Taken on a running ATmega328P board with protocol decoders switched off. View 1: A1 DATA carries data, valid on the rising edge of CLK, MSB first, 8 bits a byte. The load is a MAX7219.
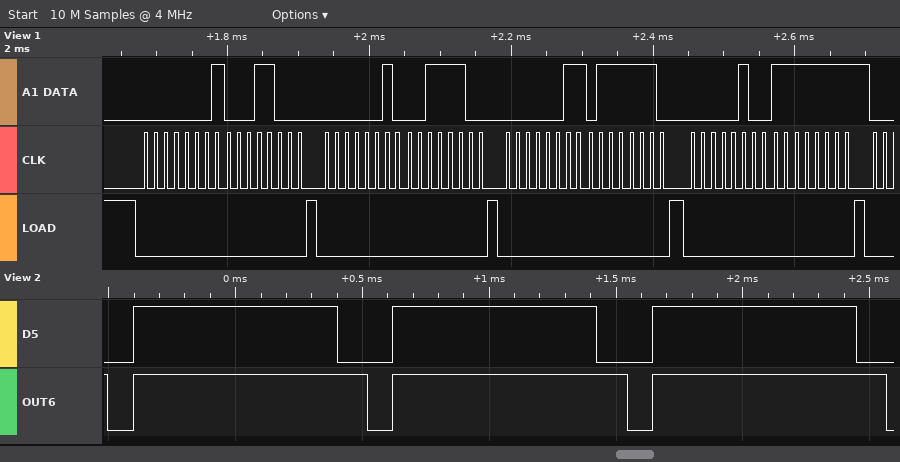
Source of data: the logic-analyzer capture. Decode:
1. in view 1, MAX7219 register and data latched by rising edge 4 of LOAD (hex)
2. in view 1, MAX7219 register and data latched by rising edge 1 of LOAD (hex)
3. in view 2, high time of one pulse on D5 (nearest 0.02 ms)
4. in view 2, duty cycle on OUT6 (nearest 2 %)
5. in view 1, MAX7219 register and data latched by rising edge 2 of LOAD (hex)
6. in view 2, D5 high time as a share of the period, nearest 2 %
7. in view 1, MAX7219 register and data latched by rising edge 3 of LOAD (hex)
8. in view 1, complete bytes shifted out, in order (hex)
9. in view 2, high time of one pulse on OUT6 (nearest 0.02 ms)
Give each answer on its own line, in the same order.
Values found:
register 0x4, data 0xFF
register 0x1, data 0x18
0.80 ms
90 %
register 0x2, data 0x3C
78 %
register 0x3, data 0x7E
0x01 0x18 0x02 0x3C 0x03 0x7E 0x04 0xFF
0.92 ms
